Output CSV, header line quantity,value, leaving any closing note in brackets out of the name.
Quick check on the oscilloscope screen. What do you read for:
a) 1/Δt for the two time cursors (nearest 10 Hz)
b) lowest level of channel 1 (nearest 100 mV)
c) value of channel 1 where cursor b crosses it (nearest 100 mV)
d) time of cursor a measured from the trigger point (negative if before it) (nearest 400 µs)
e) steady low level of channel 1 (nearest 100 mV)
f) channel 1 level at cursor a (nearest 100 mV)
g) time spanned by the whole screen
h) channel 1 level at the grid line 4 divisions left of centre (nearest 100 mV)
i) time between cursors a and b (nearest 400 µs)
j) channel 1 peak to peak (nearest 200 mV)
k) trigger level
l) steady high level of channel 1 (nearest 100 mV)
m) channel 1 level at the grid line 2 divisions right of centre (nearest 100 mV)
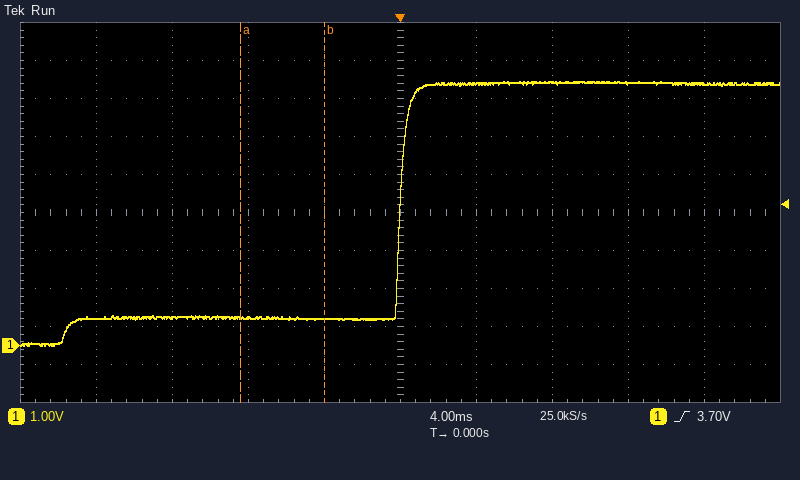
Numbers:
quantity,value
1/Δt for the two time cursors,230 Hz
lowest level of channel 1,0.0 V
value of channel 1 where cursor b crosses it,700 mV
time of cursor a measured from the trigger point (negative if before it),-8.4 ms
steady low level of channel 1,700 mV
channel 1 level at cursor a,700 mV
time spanned by the whole screen,40 ms
channel 1 level at the grid line 4 divisions left of centre,700 mV
time between cursors a and b,4.4 ms
channel 1 peak to peak,7.0 V
trigger level,3.70 V
steady high level of channel 1,6.9 V
channel 1 level at the grid line 2 divisions right of centre,6.9 V
